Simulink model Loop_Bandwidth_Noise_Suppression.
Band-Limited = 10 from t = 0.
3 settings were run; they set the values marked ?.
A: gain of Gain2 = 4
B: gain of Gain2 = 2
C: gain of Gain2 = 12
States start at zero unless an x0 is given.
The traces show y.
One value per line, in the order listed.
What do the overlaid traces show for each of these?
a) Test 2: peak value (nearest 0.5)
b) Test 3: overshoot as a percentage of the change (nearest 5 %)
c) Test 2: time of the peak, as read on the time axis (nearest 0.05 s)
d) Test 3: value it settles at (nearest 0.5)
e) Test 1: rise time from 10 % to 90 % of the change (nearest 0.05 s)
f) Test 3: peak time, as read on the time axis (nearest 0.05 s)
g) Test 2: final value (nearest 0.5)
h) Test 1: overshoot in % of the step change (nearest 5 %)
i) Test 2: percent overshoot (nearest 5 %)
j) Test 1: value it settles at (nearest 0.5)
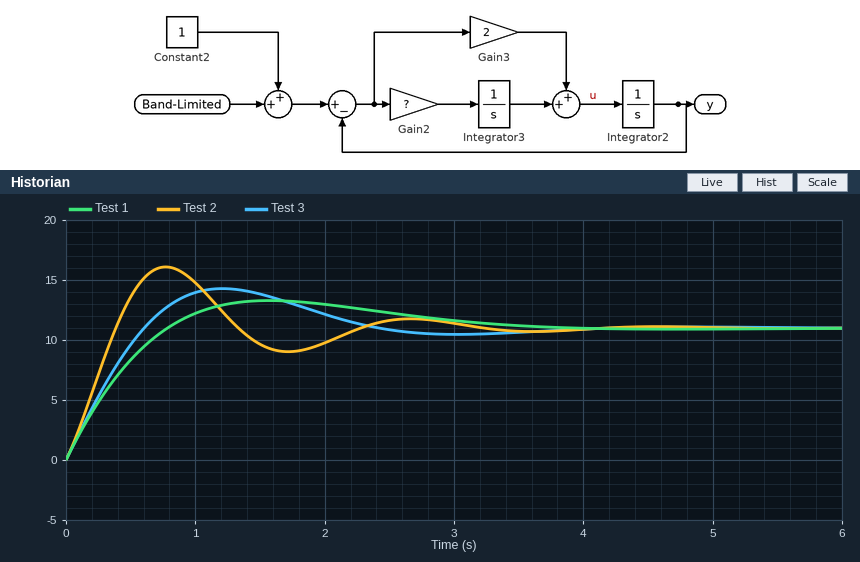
16.0
30 %
0.75 s
11.0
0.60 s
1.20 s
11.0
20 %
45 %
11.0
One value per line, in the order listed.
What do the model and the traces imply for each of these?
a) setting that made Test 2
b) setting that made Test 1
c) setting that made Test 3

C
B
A
